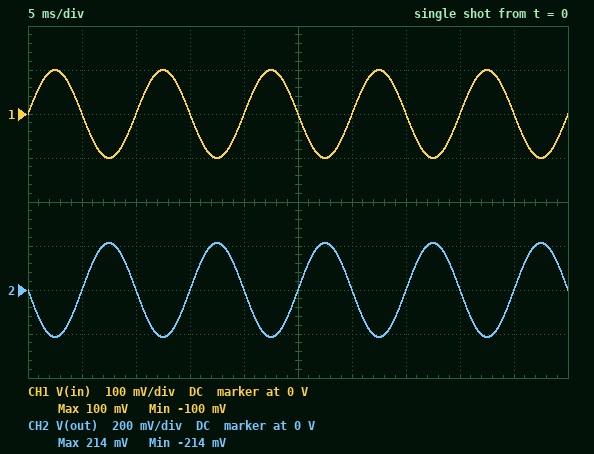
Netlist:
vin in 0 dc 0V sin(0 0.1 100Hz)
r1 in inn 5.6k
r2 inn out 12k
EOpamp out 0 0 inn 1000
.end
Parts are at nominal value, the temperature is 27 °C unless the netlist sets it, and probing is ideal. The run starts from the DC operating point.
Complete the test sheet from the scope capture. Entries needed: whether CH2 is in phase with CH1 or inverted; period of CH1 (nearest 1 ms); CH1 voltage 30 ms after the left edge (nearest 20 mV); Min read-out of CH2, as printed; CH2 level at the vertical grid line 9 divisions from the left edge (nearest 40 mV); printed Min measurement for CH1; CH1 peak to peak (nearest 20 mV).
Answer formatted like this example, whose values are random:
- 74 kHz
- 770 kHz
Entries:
- inverted
- 10 ms
- 0 V
- -214 mV
- 0 V
- -100 mV
- 200 mV
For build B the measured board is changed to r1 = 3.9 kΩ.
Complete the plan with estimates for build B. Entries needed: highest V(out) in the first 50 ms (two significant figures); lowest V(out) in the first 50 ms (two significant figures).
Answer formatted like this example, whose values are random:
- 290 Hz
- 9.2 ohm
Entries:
- 310 mV
- -310 mV
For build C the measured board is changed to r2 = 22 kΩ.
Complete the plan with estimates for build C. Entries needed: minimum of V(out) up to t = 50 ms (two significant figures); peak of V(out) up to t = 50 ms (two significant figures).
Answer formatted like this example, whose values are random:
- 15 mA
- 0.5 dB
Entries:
- -390 mV
- 390 mV
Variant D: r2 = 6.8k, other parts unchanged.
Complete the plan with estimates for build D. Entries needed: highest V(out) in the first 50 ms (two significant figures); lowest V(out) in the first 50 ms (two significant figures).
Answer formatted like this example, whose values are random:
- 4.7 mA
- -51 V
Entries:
- 120 mV
- -120 mV
